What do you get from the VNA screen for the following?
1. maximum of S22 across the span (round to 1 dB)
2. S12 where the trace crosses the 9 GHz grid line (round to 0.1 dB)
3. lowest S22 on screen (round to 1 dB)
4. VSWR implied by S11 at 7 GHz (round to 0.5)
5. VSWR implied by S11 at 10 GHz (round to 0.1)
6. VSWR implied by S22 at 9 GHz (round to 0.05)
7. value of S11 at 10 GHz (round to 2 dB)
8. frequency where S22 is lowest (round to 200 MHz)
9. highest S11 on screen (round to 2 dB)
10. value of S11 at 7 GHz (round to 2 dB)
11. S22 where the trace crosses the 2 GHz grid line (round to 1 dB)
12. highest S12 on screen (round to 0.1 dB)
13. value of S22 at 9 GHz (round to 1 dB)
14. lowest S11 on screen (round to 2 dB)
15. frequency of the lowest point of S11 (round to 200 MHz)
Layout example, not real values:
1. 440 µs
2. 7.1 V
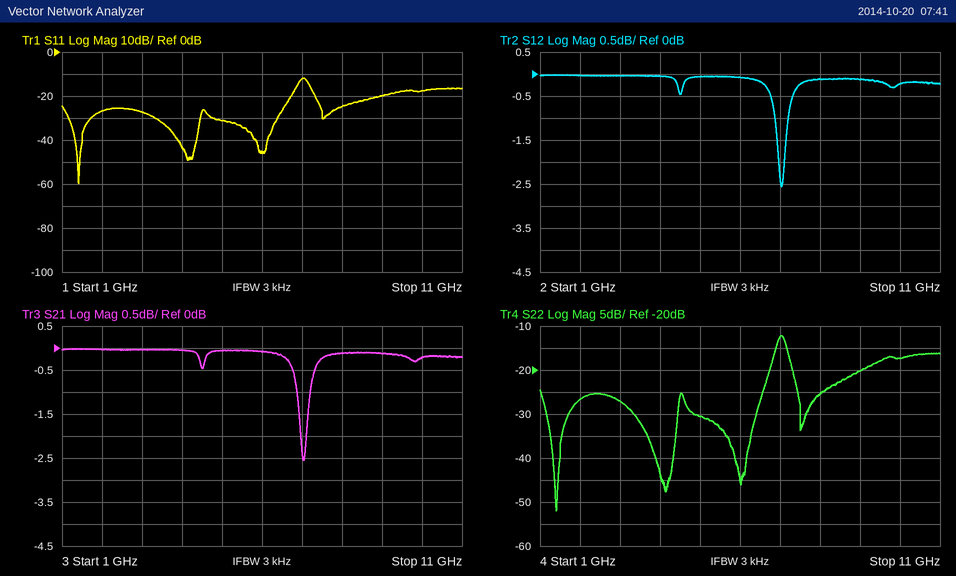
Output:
1. -12 dB
2. -0.1 dB
3. -52 dB
4. 1.5
5. 1.3
6. 1.20
7. -18 dB
8. 1.4 GHz
9. -12 dB
10. -12 dB
11. -27 dB
12. 0.0 dB
13. -20 dB
14. -60 dB
15. 1.4 GHz
